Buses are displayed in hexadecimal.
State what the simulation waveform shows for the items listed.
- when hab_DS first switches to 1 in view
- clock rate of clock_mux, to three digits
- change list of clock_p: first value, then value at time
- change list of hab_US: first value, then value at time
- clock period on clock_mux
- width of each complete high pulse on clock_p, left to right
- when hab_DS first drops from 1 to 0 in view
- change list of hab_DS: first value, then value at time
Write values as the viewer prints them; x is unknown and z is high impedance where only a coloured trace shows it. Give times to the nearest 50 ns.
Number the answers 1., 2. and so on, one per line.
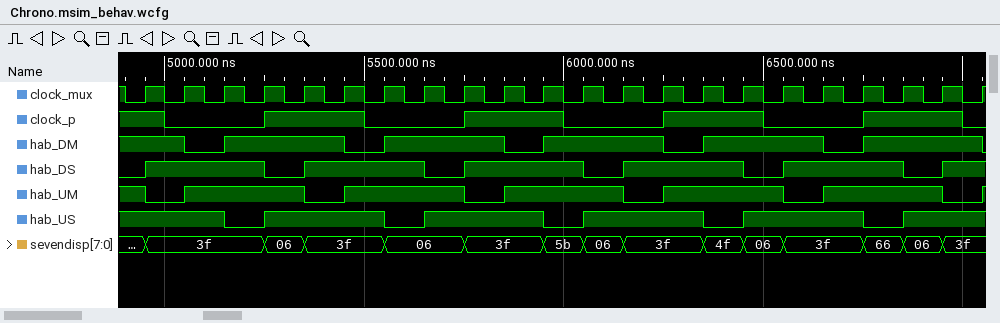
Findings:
1. 4950 ns
2. 10.0 MHz
3. 1, 0 at 5000 ns, 1 at 5250 ns, 0 at 5500 ns, 1 at 5750 ns, 0 at 6000 ns, 1 at 6250 ns, 0 at 6500 ns, 1 at 6750 ns, 0 at 7000 ns
4. 1, 0 at 5150 ns, 1 at 5250 ns, 0 at 5550 ns, 1 at 5650 ns, 0 at 5950 ns, 1 at 6050 ns, 0 at 6350 ns, 1 at 6450 ns, 0 at 6750 ns, 1 at 6850 ns
5. 100 ns
6. 250 ns, 250 ns, 250 ns, 250 ns
7. 5250 ns
8. 0, 1 at 4950 ns, 0 at 5250 ns, 1 at 5350 ns, 0 at 5650 ns, 1 at 5750 ns, 0 at 6050 ns, 1 at 6150 ns, 0 at 6450 ns, 1 at 6550 ns, 0 at 6850 ns, 1 at 6950 ns
